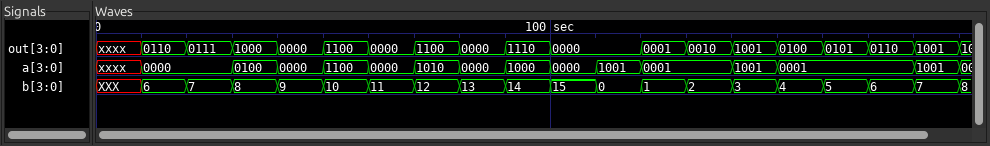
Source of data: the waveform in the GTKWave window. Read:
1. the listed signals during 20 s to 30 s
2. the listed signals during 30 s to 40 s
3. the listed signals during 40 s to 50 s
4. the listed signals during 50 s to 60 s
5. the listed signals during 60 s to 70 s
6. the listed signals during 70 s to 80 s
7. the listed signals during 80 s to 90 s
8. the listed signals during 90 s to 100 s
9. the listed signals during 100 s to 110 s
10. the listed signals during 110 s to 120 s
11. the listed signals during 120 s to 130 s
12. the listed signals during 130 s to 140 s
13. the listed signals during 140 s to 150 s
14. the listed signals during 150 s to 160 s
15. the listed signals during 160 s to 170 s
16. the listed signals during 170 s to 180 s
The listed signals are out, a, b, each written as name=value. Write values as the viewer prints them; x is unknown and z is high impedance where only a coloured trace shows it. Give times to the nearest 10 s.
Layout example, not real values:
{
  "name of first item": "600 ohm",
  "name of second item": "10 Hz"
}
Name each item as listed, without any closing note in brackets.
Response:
{
  "the listed signals during 20 s to 30 s": "out=0111, a=0000, b=7",
  "the listed signals during 30 s to 40 s": "out=1000, a=0100, b=8",
  "the listed signals during 40 s to 50 s": "out=0000, a=0000, b=9",
  "the listed signals during 50 s to 60 s": "out=1100, a=1100, b=10",
  "the listed signals during 60 s to 70 s": "out=0000, a=0000, b=11",
  "the listed signals during 70 s to 80 s": "out=1100, a=1010, b=12",
  "the listed signals during 80 s to 90 s": "out=0000, a=0000, b=13",
  "the listed signals during 90 s to 100 s": "out=1110, a=1000, b=14",
  "the listed signals during 100 s to 110 s": "out=0000, a=0000, b=15",
  "the listed signals during 110 s to 120 s": "out=0000, a=1001, b=0",
  "the listed signals during 120 s to 130 s": "out=0001, a=0001, b=1",
  "the listed signals during 130 s to 140 s": "out=0010, a=0001, b=2",
  "the listed signals during 140 s to 150 s": "out=1001, a=1001, b=3",
  "the listed signals during 150 s to 160 s": "out=0100, a=0001, b=4",
  "the listed signals during 160 s to 170 s": "out=0101, a=0001, b=5",
  "the listed signals during 170 s to 180 s": "out=0110, a=0001, b=6"
}
